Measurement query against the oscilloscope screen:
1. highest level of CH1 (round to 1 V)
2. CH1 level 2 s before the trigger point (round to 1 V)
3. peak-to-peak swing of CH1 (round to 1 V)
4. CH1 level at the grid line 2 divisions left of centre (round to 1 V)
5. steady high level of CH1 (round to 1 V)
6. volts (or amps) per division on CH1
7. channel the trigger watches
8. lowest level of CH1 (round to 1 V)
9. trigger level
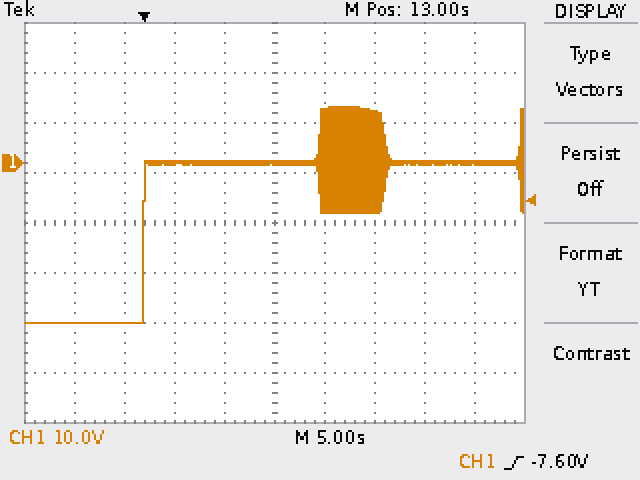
11 V
-32 V
43 V
0 V
0 V
10 V
CH1
-32 V
-7.60 V
